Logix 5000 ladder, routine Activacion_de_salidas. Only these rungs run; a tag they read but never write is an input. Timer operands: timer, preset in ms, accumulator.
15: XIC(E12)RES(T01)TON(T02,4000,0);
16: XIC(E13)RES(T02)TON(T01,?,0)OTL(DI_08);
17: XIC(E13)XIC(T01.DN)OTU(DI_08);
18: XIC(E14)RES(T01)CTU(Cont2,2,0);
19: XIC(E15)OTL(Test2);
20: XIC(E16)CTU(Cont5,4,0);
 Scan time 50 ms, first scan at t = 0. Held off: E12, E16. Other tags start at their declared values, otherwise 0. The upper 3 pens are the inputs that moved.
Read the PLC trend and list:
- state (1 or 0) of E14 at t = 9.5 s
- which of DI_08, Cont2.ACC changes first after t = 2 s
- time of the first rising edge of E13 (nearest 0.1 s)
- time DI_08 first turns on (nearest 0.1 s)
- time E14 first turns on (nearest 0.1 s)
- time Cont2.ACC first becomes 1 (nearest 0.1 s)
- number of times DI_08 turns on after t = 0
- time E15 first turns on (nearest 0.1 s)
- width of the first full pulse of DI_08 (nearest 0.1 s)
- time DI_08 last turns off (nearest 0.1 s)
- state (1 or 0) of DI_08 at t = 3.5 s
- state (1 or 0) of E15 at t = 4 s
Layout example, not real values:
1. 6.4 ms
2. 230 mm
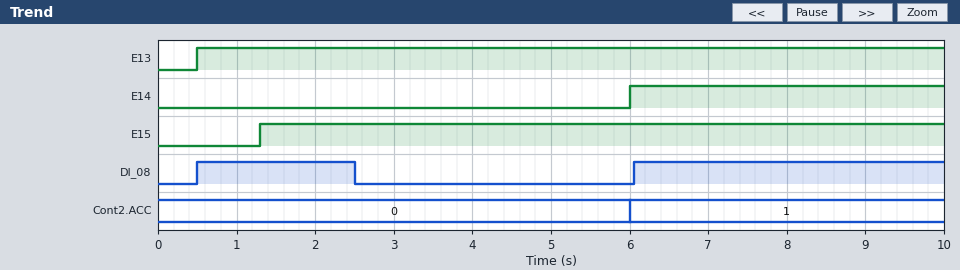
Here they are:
1. 1
2. DI_08
3. 0.5 s
4. 0.5 s
5. 6.0 s
6. 6.0 s
7. 2
8. 1.3 s
9. 2.0 s
10. 2.5 s
11. 0
12. 1
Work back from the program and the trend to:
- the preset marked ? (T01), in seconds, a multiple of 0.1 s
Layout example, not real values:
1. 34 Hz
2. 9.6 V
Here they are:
1. 2.0 s
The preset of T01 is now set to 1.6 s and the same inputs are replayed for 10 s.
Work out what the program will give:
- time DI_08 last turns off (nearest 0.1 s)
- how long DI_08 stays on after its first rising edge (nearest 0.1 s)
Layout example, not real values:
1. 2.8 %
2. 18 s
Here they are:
1. 2.1 s
2. 1.6 s
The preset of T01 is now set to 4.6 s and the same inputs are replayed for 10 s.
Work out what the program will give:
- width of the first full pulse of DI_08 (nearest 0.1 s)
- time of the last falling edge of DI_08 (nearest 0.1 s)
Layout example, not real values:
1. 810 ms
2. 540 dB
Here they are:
1. 4.6 s
2. 5.1 s
